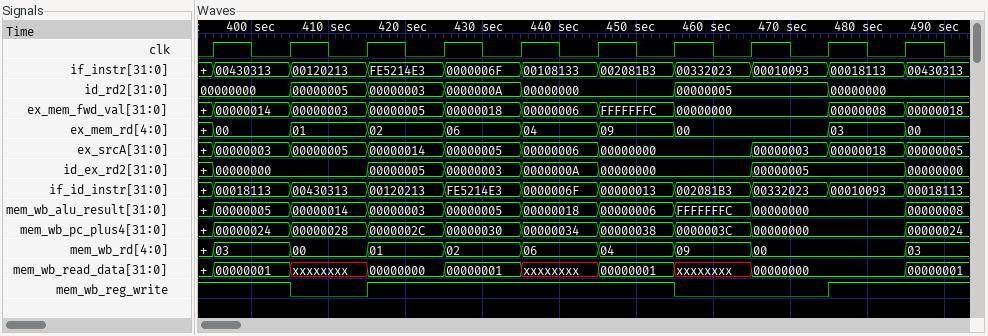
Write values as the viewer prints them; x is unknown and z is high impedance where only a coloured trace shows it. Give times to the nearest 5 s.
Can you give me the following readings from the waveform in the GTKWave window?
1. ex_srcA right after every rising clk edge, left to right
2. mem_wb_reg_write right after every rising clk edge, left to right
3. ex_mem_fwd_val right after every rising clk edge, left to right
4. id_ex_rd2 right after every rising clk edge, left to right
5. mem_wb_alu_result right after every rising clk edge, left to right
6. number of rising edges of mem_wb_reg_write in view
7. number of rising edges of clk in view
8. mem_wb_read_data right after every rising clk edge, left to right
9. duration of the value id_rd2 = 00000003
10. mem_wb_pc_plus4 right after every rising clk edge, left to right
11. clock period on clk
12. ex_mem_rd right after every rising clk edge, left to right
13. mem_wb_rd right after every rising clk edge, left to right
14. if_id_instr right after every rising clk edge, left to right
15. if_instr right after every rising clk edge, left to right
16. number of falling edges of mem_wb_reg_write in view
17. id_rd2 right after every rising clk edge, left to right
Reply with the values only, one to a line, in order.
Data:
00000003, 00000005, 00000014, 00000005, 00000006, 00000000, 00000000, 00000003, 00000018, 00000005
1 0 1 1 1 1 0 0 1 1
00000014, 00000003, 00000005, 00000018, 00000006, FFFFFFFC, 00000000, 00000000, 00000008, 00000018
00000000, 00000000, 00000005, 00000003, 0000000A, 00000000, 00000000, 00000005, 00000005, 00000000
00000005, 00000014, 00000003, 00000005, 00000018, 00000006, FFFFFFFC, 00000000, 00000000, 00000008
2
10
00000001, xxxxxxxx, 00000000, 00000001, xxxxxxxx, 00000001, xxxxxxxx, 00000000, 00000000, 00000001
10 s
00000024, 00000028, 0000002C, 00000030, 00000034, 00000038, 0000003C, 00000000, 00000000, 00000024
10 s
00, 01, 02, 06, 04, 09, 00, 00, 03, 00
03, 00, 01, 02, 06, 04, 09, 00, 00, 03
00018113, 00430313, 00120213, FE5214E3, 0000006F, 00000013, 002081B3, 00332023, 00010093, 00018113
00430313, 00120213, FE5214E3, 0000006F, 00108133, 002081B3, 00332023, 00010093, 00018113, 00430313
2
00000000, 00000005, 00000003, 0000000A, 00000000, 00000000, 00000005, 00000005, 00000000, 00000000
